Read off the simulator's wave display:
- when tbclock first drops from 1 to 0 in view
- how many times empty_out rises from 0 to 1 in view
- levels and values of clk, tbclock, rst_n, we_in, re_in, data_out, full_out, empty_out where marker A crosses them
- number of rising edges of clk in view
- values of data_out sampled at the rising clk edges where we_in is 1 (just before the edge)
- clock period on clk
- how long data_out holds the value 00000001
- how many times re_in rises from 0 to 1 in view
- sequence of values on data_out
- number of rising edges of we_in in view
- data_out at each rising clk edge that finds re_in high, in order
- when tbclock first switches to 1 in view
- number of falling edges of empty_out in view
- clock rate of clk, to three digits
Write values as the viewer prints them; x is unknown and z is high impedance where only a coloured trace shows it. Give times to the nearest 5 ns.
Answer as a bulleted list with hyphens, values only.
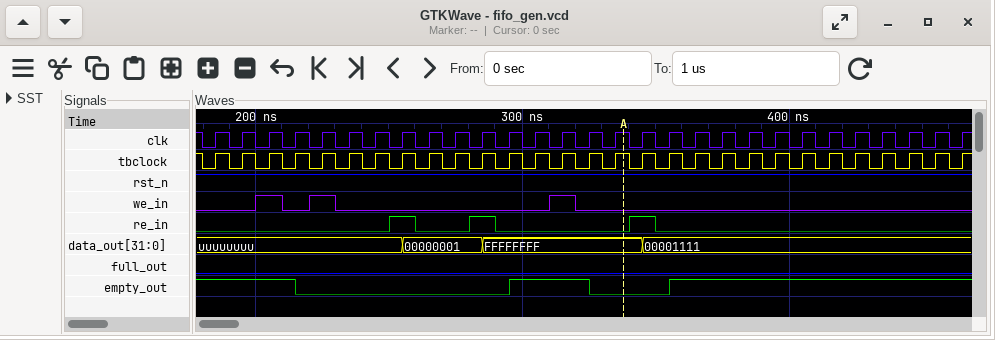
- 180 ns
- 2
- clk=1, tbclock=1, rst_n=1, we_in=0, re_in=0, data_out=FFFFFFFF, full_out=0, empty_out=0
- 29
- uuuuuuuu, uuuuuuuu, FFFFFFFF
- 10 ns
- 30 ns
- 3
- uuuuuuuu, 00000001, FFFFFFFF, 00001111
- 3
- uuuuuuuu, 00000001, FFFFFFFF
- 185 ns
- 2
- 100 MHz
